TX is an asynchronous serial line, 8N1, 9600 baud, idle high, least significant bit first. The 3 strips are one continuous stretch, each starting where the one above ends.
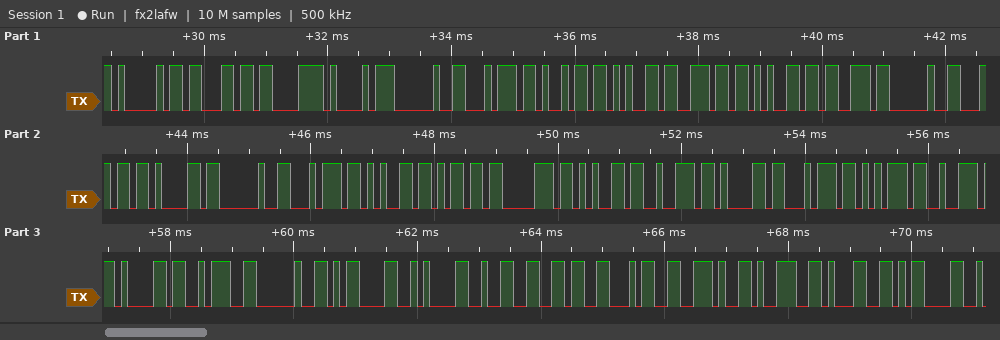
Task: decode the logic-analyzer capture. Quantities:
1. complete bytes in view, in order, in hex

41 63 C3 A1 20 74 69 65 6E 65 73 20 6C 61 20 74 65 6D 70 65 72 61 74 75 72 61 3A 20 0D 0A 32 36 34 2E 39 31 0D
